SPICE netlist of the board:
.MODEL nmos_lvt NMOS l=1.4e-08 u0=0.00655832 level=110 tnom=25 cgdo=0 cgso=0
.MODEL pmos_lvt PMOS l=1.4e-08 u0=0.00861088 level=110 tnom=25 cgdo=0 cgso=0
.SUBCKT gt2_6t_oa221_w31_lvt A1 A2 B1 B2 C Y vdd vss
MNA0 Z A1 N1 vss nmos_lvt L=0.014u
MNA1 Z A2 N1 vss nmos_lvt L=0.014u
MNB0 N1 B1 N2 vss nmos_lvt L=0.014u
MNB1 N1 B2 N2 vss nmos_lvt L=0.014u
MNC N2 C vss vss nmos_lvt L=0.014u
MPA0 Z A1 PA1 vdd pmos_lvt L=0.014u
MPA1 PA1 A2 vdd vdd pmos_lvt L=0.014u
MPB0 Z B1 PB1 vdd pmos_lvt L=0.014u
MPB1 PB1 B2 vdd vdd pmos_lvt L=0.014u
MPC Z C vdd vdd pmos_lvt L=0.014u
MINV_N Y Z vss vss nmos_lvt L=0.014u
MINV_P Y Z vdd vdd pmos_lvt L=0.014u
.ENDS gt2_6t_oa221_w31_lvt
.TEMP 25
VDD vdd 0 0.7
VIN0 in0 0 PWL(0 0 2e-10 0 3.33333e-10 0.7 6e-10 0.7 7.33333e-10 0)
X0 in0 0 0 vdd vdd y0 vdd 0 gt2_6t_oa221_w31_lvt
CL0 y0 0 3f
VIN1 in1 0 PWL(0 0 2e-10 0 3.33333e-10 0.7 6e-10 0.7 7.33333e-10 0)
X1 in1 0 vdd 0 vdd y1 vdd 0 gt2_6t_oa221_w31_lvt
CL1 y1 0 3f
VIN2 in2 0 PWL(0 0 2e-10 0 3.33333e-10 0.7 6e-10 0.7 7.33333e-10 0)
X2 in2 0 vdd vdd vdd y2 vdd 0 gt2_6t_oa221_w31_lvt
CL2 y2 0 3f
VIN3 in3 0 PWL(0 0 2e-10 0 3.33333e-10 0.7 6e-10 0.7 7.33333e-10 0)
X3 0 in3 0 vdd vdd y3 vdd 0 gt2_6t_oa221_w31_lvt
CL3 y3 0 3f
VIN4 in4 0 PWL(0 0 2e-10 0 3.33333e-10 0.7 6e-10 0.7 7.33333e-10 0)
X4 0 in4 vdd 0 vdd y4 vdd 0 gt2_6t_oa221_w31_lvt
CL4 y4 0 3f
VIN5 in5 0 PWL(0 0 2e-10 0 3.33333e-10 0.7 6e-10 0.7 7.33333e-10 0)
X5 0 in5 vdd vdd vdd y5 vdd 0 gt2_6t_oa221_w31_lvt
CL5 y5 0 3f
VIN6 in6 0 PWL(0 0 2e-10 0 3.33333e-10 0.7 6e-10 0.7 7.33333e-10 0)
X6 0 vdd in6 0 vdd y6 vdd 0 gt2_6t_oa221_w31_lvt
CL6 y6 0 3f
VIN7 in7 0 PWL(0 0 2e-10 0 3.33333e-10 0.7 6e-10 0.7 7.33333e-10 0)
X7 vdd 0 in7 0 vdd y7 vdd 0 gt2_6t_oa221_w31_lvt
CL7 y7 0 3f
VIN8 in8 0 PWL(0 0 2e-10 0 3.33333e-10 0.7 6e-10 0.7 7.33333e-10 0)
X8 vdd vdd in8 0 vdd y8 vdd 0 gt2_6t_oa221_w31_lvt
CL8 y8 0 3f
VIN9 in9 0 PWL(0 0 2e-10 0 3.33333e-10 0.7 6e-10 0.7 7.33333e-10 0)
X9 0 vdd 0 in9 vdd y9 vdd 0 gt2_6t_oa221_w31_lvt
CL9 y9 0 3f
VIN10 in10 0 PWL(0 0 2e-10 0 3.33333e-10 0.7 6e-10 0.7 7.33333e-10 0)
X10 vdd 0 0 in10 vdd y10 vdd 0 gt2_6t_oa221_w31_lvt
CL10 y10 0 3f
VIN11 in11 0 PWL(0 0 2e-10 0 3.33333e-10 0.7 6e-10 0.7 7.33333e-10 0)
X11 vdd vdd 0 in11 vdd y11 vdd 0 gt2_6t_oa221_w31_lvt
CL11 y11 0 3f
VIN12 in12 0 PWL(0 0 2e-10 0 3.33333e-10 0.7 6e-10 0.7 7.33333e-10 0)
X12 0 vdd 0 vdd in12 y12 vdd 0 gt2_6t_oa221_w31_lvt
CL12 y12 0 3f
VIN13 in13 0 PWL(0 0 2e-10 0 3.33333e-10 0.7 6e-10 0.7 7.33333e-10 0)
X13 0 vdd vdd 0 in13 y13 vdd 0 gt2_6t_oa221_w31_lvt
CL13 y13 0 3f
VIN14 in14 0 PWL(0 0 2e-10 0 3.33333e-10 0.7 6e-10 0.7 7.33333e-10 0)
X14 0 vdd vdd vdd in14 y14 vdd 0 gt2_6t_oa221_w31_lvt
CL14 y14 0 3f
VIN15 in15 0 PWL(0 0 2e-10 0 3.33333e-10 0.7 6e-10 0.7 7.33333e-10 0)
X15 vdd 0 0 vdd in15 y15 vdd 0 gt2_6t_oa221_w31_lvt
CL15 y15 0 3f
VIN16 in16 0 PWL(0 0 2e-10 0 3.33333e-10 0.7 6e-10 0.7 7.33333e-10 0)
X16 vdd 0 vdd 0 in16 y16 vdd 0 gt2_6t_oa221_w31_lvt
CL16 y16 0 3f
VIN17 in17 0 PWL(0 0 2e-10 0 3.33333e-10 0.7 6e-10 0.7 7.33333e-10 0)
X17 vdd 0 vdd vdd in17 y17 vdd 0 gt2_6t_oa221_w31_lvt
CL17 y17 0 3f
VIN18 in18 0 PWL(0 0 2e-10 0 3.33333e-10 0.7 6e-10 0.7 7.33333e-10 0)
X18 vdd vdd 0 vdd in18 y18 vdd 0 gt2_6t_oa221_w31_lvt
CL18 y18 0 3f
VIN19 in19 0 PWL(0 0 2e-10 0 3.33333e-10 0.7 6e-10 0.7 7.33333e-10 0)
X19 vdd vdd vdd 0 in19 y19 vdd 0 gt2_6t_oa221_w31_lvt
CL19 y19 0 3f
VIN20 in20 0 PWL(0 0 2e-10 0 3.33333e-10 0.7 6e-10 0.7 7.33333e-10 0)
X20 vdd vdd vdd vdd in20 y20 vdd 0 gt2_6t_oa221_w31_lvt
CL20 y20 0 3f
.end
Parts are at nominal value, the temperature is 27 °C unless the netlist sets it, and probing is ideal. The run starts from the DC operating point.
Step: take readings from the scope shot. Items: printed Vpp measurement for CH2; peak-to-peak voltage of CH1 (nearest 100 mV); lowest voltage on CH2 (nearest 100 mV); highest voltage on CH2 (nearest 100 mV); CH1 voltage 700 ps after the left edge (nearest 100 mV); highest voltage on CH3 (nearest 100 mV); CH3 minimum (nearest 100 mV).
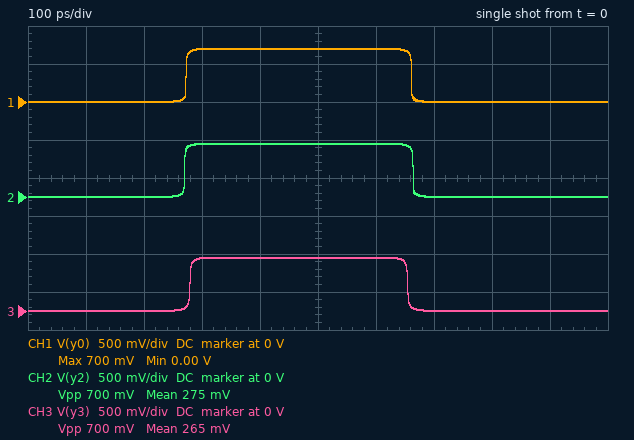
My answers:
700 mV
700 mV
0 V
700 mV
0 V
700 mV
0 V
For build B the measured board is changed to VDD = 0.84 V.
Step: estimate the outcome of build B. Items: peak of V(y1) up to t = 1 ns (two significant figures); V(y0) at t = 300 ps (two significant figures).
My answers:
840 mV
810 mV
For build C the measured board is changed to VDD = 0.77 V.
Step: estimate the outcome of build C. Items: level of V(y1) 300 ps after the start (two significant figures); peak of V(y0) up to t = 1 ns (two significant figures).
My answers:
760 mV
770 mV
